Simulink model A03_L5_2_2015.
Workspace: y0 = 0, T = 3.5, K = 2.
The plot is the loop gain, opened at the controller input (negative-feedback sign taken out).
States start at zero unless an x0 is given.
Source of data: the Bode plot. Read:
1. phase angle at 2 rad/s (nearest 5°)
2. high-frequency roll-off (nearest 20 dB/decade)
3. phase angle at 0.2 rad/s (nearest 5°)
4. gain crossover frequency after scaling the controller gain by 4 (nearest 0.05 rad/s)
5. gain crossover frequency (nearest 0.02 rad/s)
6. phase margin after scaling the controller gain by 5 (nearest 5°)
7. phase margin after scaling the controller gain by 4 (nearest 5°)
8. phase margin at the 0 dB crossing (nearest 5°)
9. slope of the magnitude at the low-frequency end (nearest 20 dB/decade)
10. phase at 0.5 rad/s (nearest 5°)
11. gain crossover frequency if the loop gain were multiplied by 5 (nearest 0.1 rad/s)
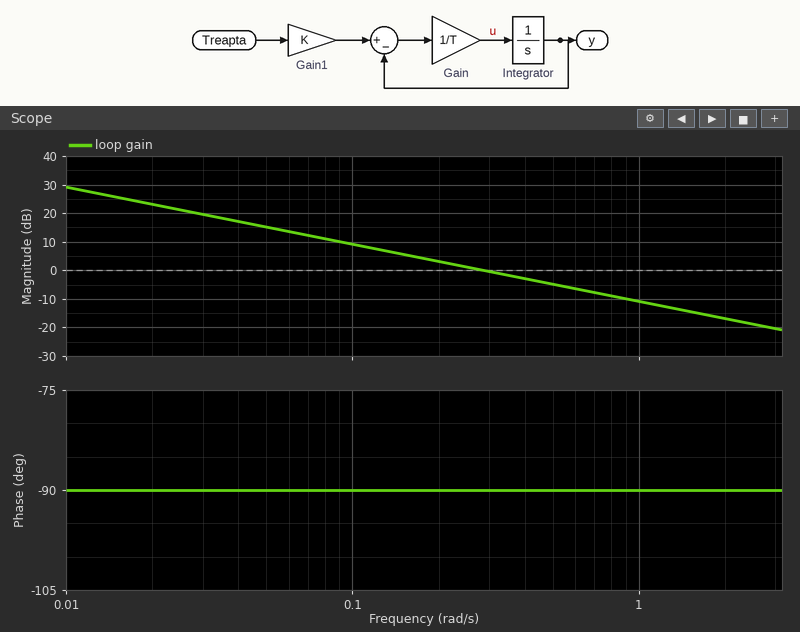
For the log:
-90°
-20 dB/decade
-90°
1.15 rad/s
0.28 rad/s
90°
90°
90°
-20 dB/decade
-90°
1.4 rad/s
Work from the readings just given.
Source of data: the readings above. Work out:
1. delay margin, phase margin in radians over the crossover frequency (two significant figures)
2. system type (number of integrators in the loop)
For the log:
5.6 s
1
